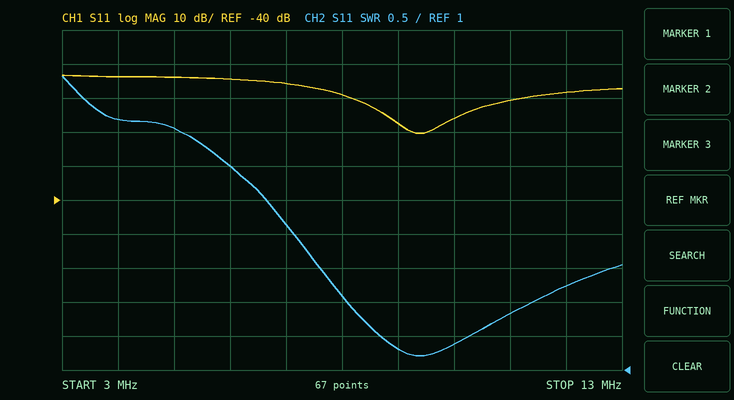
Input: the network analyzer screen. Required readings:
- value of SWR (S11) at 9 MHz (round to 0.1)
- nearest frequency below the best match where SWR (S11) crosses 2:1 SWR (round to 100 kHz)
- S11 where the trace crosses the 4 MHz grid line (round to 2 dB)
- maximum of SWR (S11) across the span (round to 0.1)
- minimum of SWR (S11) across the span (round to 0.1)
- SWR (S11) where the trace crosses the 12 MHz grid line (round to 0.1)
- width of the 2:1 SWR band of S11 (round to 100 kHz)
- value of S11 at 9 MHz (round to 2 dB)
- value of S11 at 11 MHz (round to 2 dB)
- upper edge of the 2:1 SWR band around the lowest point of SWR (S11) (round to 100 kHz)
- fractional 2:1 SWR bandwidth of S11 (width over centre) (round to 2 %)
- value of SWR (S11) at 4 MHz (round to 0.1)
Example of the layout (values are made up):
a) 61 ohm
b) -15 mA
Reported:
a) 1.3
b) 8.1 MHz
c) -4 dB
d) 5.3
e) 1.2
f) 2.2
g) 3.3 MHz
h) -18 dB
i) -10 dB
j) 11.4 MHz
k) 34 %
l) 4.7
